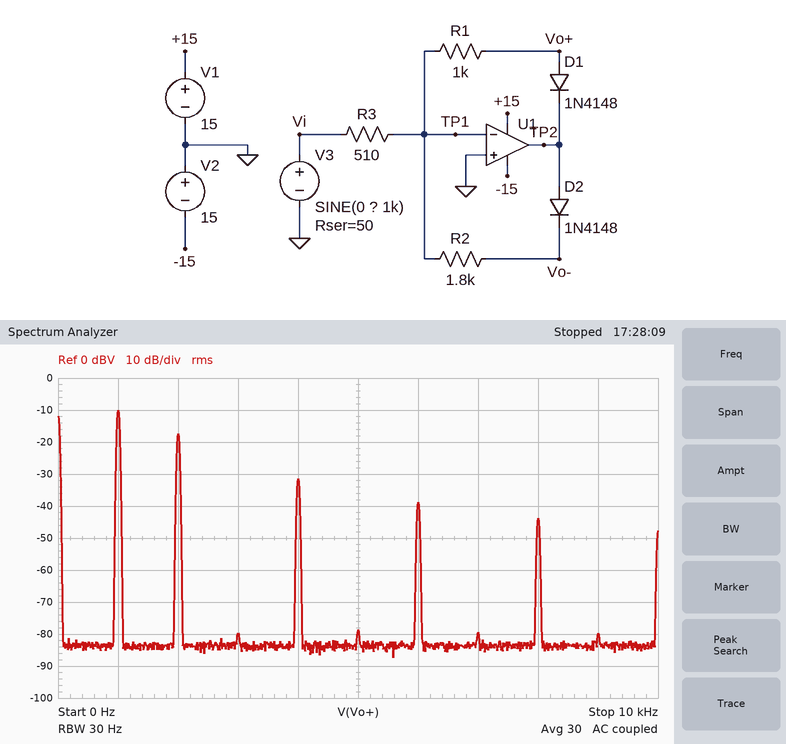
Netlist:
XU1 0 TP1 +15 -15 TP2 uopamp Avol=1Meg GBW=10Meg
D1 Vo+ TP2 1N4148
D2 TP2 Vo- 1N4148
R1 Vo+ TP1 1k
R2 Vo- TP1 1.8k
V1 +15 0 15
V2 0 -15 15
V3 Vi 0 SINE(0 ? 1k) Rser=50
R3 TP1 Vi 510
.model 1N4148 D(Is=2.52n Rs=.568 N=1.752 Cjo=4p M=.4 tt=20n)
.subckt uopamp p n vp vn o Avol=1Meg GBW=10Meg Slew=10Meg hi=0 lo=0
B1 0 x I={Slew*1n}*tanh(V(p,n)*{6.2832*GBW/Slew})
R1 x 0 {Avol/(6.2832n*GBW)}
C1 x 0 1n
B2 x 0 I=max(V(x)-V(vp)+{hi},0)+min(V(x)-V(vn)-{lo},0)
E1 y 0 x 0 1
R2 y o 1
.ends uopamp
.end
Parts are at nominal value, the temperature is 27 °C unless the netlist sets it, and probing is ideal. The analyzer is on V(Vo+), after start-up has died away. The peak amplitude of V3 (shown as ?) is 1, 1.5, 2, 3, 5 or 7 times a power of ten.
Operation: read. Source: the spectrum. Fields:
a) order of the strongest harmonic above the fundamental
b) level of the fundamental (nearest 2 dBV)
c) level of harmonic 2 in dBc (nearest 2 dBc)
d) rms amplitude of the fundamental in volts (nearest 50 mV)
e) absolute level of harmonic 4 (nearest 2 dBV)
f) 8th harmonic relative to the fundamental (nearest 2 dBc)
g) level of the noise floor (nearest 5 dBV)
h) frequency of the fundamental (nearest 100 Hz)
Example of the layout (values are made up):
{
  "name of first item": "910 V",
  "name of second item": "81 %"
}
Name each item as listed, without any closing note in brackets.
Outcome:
{
  "order of the strongest harmonic above the fundamental": "2",
  "level of the fundamental": "-10 dBV",
  "level of harmonic 2 in dBc": "-8 dBc",
  "rms amplitude of the fundamental in volts": "300 mV",
  "absolute level of harmonic 4": "-32 dBV",
  "8th harmonic relative to the fundamental": "-34 dBc",
  "level of the noise floor": "-85 dBV",
  "frequency of the fundamental": "1.0 kHz"
}
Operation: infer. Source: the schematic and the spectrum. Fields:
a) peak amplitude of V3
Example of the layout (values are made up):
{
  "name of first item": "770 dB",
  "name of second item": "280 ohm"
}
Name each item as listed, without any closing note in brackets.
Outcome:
{
  "peak amplitude of V3": "500 mV"
}
